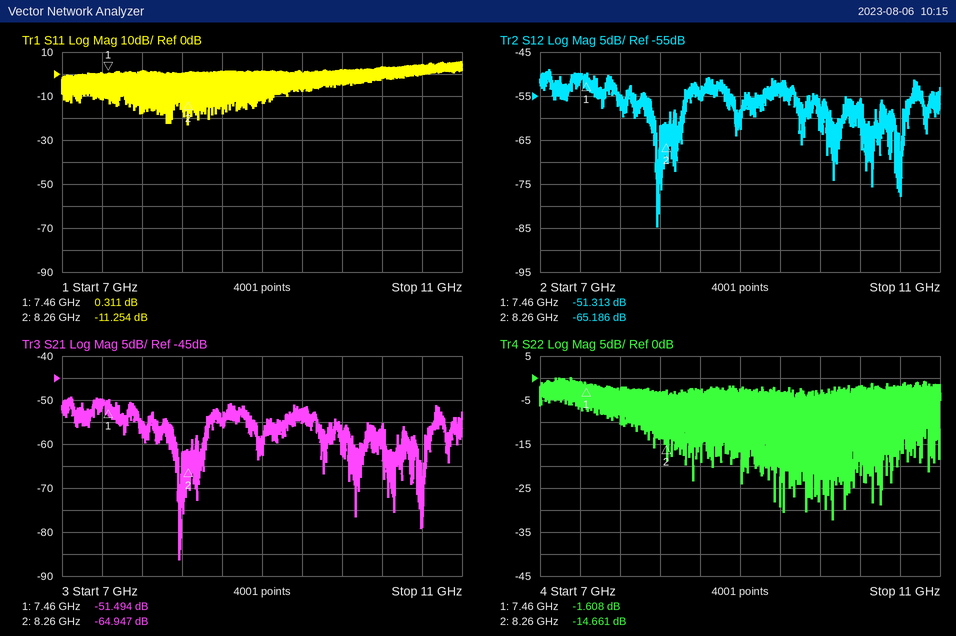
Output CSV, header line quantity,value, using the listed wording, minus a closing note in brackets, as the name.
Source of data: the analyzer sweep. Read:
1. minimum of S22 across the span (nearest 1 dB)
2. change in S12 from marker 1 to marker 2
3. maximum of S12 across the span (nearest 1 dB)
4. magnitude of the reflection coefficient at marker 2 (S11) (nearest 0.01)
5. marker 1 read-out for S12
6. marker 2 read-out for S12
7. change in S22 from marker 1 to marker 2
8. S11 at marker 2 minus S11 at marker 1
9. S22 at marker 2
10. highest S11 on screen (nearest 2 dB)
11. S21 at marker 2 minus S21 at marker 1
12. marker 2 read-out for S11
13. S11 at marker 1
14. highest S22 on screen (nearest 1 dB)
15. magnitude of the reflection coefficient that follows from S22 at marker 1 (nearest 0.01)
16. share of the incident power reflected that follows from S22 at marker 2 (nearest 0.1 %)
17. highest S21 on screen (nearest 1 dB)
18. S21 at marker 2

quantity,value
minimum of S22 across the span,-32 dB
change in S12 from marker 1 to marker 2,-13.873 dB
maximum of S12 across the span,-49 dB
magnitude of the reflection coefficient at marker 2 (S11),0.27
marker 1 read-out for S12,-51.313 dB
marker 2 read-out for S12,-65.186 dB
change in S22 from marker 1 to marker 2,-13.053 dB
S11 at marker 2 minus S11 at marker 1,-11.565 dB
S22 at marker 2,-14.661 dB
highest S11 on screen,6 dB
S21 at marker 2 minus S21 at marker 1,-13.453 dB
marker 2 read-out for S11,-11.254 dB
S11 at marker 1,0.311 dB
highest S22 on screen,0 dB
magnitude of the reflection coefficient that follows from S22 at marker 1,0.83
share of the incident power reflected that follows from S22 at marker 2,3.4 %
highest S21 on screen,-49 dB
S21 at marker 2,-64.947 dB
